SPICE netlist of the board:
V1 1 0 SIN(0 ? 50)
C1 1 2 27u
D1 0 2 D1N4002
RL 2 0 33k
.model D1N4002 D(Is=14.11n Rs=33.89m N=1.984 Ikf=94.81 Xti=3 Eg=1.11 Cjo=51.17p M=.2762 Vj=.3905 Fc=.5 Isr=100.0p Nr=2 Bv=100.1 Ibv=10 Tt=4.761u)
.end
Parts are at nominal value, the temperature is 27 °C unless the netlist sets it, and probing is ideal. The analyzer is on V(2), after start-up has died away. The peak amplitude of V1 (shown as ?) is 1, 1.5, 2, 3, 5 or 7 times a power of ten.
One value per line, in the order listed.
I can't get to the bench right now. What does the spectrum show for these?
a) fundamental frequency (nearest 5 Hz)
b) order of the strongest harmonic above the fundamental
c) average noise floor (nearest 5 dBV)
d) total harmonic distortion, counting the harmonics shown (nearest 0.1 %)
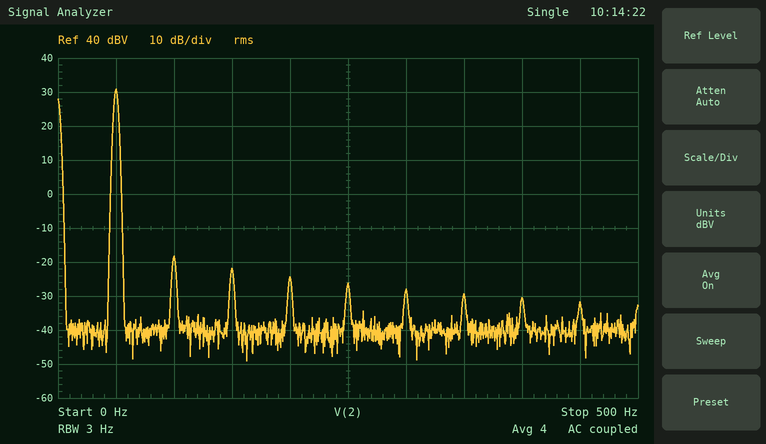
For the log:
50 Hz
2
-40 dBV
0.4 %
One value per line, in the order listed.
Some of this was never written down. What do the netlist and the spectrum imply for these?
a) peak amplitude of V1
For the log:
50 V
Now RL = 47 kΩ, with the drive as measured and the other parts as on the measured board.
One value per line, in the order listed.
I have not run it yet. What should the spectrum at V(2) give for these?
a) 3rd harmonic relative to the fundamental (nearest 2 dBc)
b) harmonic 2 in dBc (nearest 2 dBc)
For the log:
-56 dBc
-52 dBc
